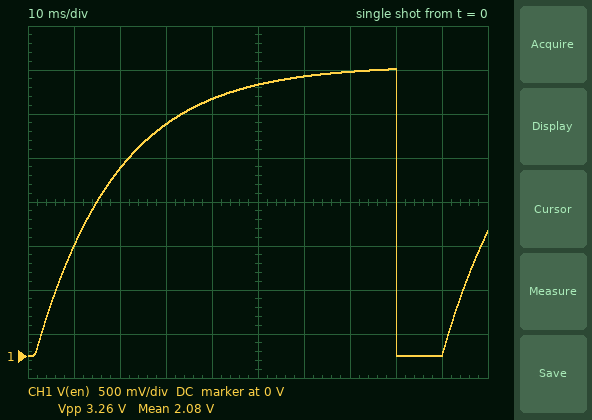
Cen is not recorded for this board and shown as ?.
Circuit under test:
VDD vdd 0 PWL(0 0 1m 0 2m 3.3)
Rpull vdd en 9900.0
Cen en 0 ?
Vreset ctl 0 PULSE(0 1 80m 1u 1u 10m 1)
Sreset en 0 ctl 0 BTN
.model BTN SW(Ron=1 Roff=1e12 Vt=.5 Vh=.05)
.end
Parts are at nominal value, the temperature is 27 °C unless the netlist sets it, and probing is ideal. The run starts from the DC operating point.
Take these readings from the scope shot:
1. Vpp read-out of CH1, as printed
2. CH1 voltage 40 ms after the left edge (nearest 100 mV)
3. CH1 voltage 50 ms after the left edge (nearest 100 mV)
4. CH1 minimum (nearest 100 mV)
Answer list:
3.26 V
2.9 V
3.1 V
0 V
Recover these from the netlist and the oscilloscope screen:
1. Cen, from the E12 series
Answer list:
1.8 µF
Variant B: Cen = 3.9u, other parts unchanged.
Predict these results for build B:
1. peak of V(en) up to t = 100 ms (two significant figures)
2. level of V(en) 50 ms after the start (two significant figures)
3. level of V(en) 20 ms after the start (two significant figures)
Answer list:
2.9 V
2.4 V
1.3 V
